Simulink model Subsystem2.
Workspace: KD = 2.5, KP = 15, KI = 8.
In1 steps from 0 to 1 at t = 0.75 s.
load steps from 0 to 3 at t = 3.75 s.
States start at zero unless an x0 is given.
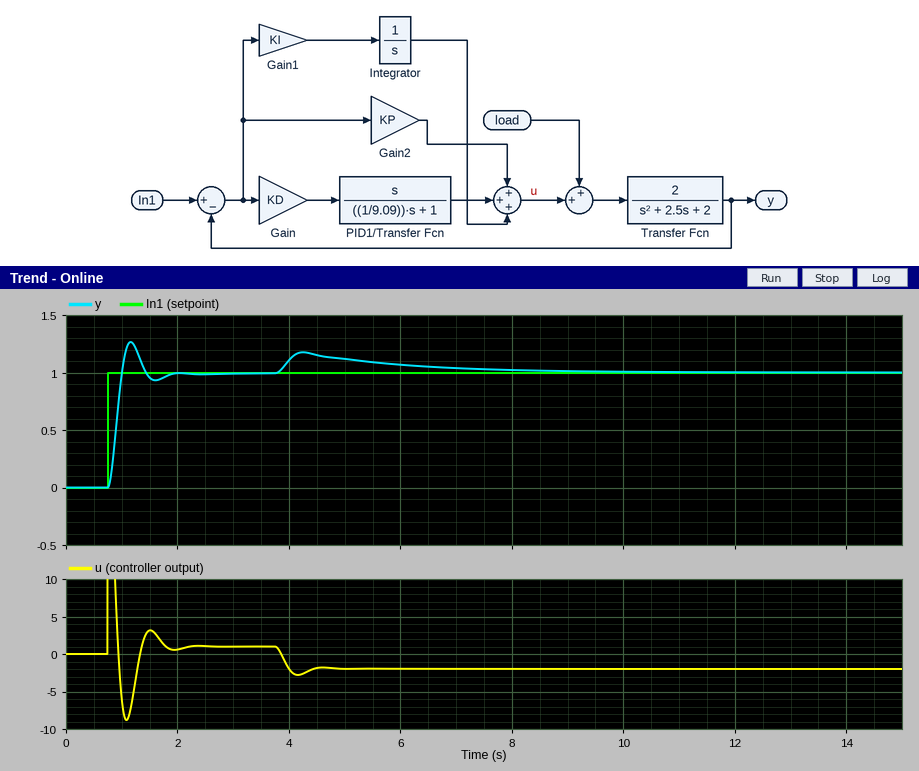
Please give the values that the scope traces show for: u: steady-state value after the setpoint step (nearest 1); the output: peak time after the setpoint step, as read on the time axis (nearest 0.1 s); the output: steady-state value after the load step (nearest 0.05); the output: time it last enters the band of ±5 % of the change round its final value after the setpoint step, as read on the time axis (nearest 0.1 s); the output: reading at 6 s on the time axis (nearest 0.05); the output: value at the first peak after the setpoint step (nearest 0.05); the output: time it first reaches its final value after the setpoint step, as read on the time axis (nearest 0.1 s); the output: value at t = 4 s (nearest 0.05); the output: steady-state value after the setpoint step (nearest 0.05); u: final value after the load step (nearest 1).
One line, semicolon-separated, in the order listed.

1; 1.2 s; 1.00; 1.7 s; 1.05; 1.25; 1.0 s; 1.10; 1.00; -2
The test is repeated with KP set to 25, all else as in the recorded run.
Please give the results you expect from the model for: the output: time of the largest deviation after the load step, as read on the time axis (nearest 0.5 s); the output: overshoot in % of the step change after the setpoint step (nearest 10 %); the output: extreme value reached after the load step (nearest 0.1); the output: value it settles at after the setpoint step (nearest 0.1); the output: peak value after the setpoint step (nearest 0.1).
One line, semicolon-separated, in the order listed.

4.0 s; 40 %; 1.1; 1.0; 1.4
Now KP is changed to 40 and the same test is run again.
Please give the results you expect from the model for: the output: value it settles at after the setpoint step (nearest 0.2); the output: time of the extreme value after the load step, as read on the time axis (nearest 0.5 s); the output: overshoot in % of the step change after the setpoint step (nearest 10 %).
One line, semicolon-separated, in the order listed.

1.0; 4.0 s; 50 %
